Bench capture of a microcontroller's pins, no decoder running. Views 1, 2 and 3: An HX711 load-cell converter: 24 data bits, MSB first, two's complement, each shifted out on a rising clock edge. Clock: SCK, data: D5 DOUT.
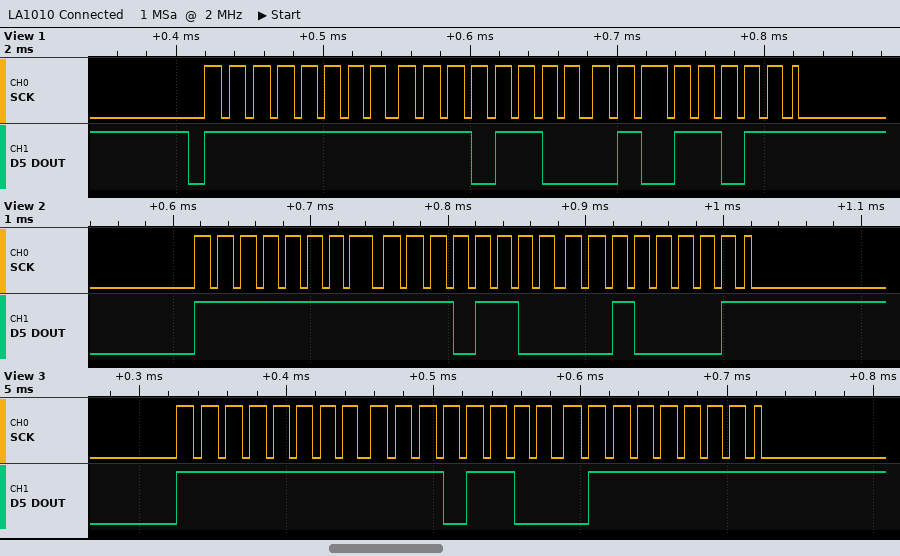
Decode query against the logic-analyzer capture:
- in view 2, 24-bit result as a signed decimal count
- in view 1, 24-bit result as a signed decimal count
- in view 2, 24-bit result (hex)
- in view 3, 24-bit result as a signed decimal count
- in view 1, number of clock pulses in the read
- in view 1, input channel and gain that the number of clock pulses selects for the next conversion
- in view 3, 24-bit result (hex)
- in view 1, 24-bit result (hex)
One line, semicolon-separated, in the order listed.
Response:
-5087; -5029; 0xFFEC21; -4993; 25; channel A, gain 128; 0xFFEC7F; 0xFFEC5B
